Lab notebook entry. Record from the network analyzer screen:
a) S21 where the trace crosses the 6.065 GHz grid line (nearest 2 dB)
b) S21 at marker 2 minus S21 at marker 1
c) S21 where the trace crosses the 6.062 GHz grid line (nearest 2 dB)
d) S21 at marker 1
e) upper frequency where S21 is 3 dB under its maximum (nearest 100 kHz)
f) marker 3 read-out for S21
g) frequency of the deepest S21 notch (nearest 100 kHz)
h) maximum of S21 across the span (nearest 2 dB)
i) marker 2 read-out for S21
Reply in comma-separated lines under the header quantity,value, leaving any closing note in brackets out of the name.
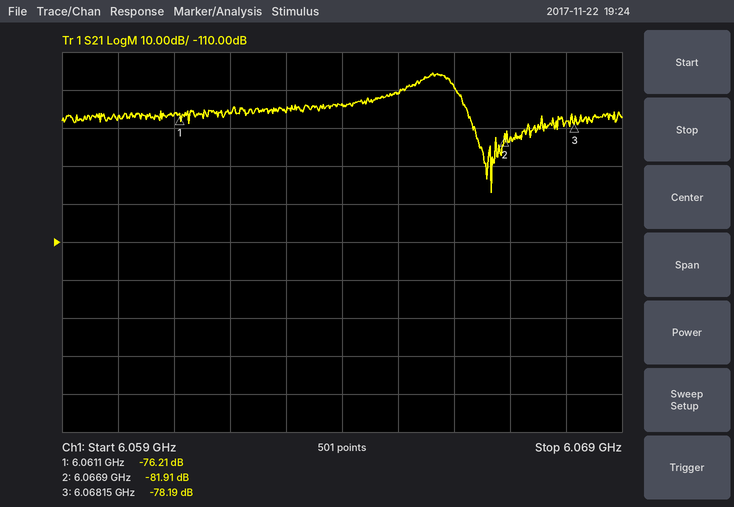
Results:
quantity,value
S21 where the trace crosses the 6.065 GHz grid line,-70 dB
S21 at marker 2 minus S21 at marker 1,-5.70 dB
S21 where the trace crosses the 6.062 GHz grid line,-76 dB
S21 at marker 1,-76.21 dB
upper frequency where S21 is 3 dB under its maximum,6.0660 GHz
marker 3 read-out for S21,-78.19 dB
frequency of the deepest S21 notch,6.0667 GHz
maximum of S21 across the span,-66 dB
marker 2 read-out for S21,-81.91 dB
